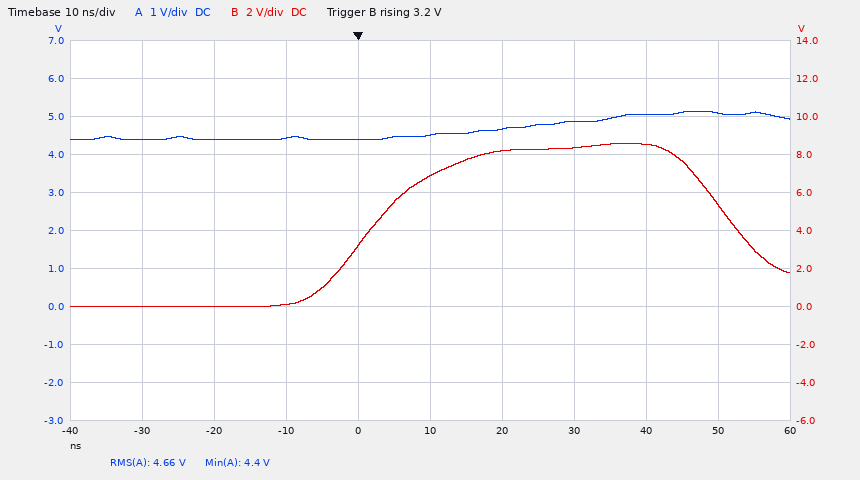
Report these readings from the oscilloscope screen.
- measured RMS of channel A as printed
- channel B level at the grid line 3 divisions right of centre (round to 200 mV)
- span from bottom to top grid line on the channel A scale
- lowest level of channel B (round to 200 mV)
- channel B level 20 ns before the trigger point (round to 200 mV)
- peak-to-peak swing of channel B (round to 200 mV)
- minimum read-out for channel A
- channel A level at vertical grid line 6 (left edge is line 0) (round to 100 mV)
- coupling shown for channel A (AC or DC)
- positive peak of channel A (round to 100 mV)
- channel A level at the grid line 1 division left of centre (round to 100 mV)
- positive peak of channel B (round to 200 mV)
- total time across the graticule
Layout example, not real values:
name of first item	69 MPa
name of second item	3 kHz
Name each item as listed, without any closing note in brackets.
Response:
measured RMS of channel A as printed	4.66 V
channel B level at the grid line 3 divisions right of centre	8.6 V
span from bottom to top grid line on the channel A scale	10 V
lowest level of channel B	0.0 V
channel B level 20 ns before the trigger point	0.0 V
peak-to-peak swing of channel B	8.6 V
minimum read-out for channel A	4.4 V
channel A level at vertical grid line 6 (left edge is line 0)	4.7 V
coupling shown for channel A	DC
positive peak of channel A	5.1 V
channel A level at the grid line 1 division left of centre	4.4 V
positive peak of channel B	8.6 V
total time across the graticule	100 ns
